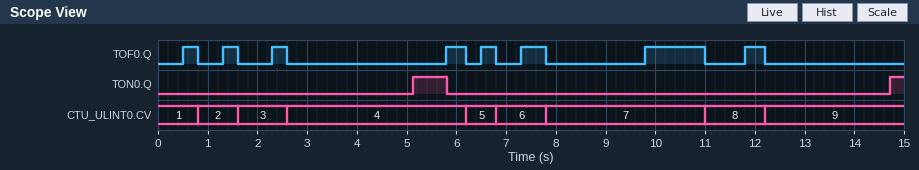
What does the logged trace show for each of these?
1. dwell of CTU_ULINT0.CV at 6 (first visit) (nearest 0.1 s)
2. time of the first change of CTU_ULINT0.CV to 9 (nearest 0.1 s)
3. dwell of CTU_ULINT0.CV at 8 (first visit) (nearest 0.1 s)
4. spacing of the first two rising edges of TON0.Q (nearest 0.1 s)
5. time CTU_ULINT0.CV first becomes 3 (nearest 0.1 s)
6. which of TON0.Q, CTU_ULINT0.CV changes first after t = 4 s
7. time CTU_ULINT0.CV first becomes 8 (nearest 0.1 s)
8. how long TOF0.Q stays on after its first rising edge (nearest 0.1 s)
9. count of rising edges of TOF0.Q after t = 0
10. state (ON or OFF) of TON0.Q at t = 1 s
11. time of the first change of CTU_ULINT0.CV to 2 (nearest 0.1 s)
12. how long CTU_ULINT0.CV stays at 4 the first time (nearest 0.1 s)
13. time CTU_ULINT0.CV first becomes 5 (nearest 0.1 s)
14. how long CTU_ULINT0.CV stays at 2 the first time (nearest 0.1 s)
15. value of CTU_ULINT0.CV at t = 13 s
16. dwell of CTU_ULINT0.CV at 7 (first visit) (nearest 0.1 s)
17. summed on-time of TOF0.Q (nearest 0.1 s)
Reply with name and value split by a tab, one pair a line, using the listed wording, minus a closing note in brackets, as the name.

dwell of CTU_ULINT0.CV at 6 (first visit)	1.0 s
time of the first change of CTU_ULINT0.CV to 9	12.2 s
dwell of CTU_ULINT0.CV at 8 (first visit)	1.2 s
spacing of the first two rising edges of TON0.Q	9.6 s
time CTU_ULINT0.CV first becomes 3	1.6 s
which of TON0.Q, CTU_ULINT0.CV changes first after t = 4 s	TON0.Q
time CTU_ULINT0.CV first becomes 8	11.0 s
how long TOF0.Q stays on after its first rising edge	0.3 s
count of rising edges of TOF0.Q after t = 0	8
state (ON or OFF) of TON0.Q at t = 1 s	OFF
time of the first change of CTU_ULINT0.CV to 2	0.8 s
how long CTU_ULINT0.CV stays at 4 the first time	3.6 s
time CTU_ULINT0.CV first becomes 5	6.2 s
how long CTU_ULINT0.CV stays at 2 the first time	0.8 s
value of CTU_ULINT0.CV at t = 13 s	9
dwell of CTU_ULINT0.CV at 7 (first visit)	3.2 s
summed on-time of TOF0.Q	3.7 s
